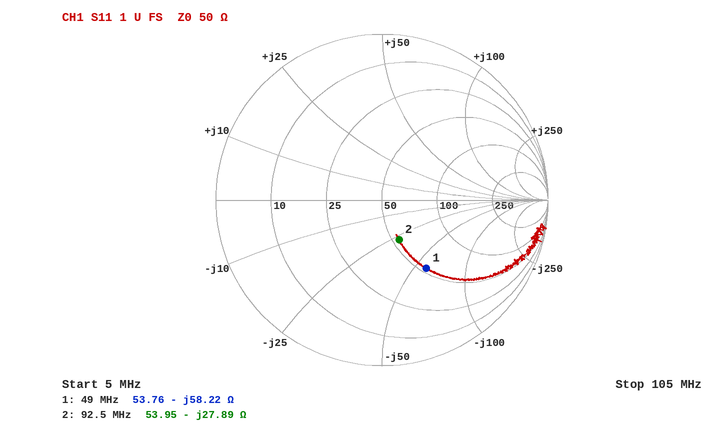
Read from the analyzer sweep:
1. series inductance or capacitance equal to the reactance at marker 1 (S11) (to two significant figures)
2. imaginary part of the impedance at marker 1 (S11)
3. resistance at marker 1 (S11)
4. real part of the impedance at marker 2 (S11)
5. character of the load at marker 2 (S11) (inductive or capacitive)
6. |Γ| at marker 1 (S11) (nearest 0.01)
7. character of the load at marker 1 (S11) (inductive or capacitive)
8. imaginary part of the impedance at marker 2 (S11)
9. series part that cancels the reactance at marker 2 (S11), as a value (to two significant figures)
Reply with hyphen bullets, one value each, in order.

- 56 pF
- -58.22 Ω
- 53.76 Ω
- 53.95 Ω
- capacitive
- 0.49
- capacitive
- -27.89 Ω
- 48 nH
